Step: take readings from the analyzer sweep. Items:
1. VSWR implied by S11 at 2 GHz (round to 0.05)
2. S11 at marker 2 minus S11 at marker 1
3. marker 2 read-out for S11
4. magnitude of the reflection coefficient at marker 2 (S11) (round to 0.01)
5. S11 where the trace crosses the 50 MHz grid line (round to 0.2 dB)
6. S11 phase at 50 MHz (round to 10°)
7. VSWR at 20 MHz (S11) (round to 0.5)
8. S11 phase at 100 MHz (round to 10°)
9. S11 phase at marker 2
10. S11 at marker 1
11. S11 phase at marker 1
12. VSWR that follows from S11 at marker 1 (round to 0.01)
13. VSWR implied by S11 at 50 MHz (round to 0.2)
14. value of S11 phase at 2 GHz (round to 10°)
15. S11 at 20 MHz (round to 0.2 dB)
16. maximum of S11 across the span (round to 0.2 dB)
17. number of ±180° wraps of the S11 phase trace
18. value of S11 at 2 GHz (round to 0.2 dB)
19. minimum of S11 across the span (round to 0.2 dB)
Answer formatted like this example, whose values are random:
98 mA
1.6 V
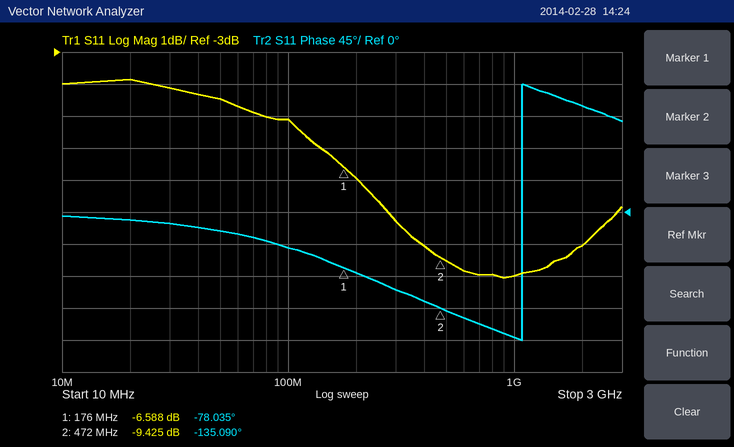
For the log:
2.10
-2.837 dB
-9.425 dB
0.34
-4.4 dB
-30°
4.5
-50°
-135.090°
-6.588 dB
-78.035°
2.76
4.0
150°
-3.8 dB
-3.8 dB
1
-9.0 dB
-10.0 dB
